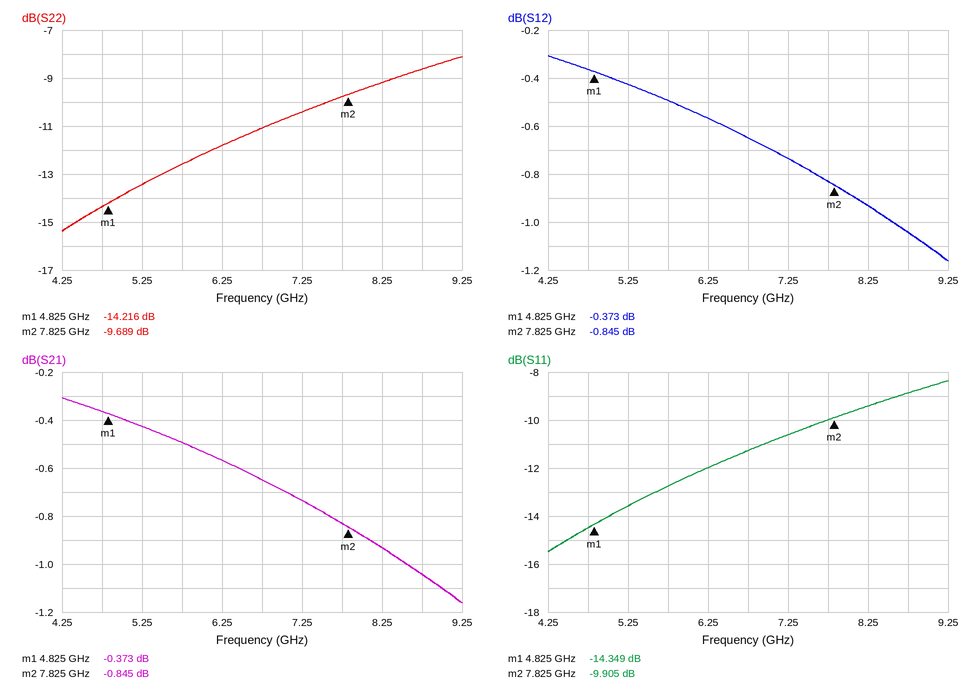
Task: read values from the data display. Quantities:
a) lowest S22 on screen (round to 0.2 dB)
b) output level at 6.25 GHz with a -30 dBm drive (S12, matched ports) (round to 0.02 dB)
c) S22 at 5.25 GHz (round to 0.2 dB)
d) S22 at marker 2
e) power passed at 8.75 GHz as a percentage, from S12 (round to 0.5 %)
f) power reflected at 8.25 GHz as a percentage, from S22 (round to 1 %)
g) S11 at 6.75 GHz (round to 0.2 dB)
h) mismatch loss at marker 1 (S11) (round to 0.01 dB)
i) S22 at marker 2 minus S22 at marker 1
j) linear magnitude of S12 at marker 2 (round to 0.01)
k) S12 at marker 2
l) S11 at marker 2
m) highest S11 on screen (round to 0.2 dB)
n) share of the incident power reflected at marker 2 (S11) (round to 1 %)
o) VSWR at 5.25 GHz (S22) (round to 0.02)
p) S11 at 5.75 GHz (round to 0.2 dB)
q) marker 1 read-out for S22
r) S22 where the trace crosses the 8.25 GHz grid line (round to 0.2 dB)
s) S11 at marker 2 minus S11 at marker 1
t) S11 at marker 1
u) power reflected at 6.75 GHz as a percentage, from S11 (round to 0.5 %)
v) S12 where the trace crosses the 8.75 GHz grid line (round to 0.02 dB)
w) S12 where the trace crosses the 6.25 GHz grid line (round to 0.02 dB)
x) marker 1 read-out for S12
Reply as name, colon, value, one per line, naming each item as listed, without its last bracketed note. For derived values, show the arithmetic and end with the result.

lowest S22 on screen: -15.4 dB
output level at 6.25 GHz with a -30 dBm drive (S12, matched ports): -30 dBm + (-0.56 dB) = -30.56 dBm
S22 at 5.25 GHz: -13.4 dB
S22 at marker 2: -9.689 dB
power passed at 8.75 GHz as a percentage, from S12: 10^(-1.04/10) ≈ 78.7 %, so 78.5 % to the nearest 0.5 %
power reflected at 8.25 GHz as a percentage, from S22: 10^(-9.2/10) ≈ 12 %
S11 at 6.75 GHz: -11.2 dB
mismatch loss at marker 1 (S11): −10 log10(1 − 10^(-14.349/10)) ≈ 0.16 dB
S22 at marker 2 minus S22 at marker 1: -9.689 − (-14.216) = 4.527 dB
linear magnitude of S12 at marker 2: 10^(-0.845/20) ≈ 0.91
S12 at marker 2: -0.845 dB
S11 at marker 2: -9.905 dB
highest S11 on screen: -8.4 dB
share of the incident power reflected at marker 2 (S11): 10^(-9.905/10) ≈ 10 %
VSWR at 5.25 GHz (S22): |Γ| = 10^(-13.4/20) = 0.2138; VSWR = (1 + 0.2138)/(1 − 0.2138) ≈ 1.54
S11 at 5.75 GHz: -12.8 dB
marker 1 read-out for S22: -14.216 dB
S22 where the trace crosses the 8.25 GHz grid line: -9.2 dB
S11 at marker 2 minus S11 at marker 1: -9.905 − (-14.349) = 4.444 dB
S11 at marker 1: -14.349 dB
power reflected at 6.75 GHz as a percentage, from S11: 10^(-11.2/10) ≈ 7.59 %, so 7.5 % to the nearest 0.5 %
S12 where the trace crosses the 8.75 GHz grid line: -1.04 dB
S12 where the trace crosses the 6.25 GHz grid line: -0.56 dB
marker 1 read-out for S12: -0.373 dB
